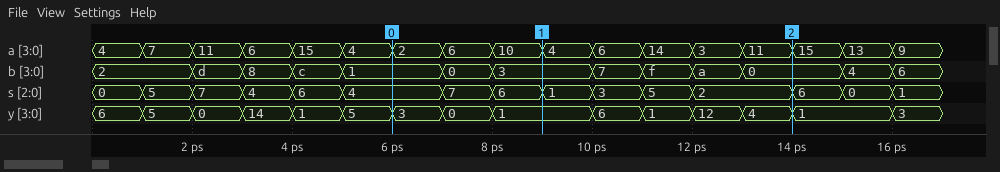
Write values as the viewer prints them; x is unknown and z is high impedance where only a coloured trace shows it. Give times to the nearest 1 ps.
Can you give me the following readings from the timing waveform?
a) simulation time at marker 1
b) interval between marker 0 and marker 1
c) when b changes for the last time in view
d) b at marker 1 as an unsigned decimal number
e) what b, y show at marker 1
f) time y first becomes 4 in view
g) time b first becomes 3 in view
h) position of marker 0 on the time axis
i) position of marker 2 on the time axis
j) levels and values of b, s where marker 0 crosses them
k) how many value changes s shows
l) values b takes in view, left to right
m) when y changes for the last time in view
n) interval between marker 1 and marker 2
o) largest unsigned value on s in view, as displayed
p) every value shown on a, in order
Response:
9 ps
3 ps
16 ps
3
b=3, y=1
13 ps
8 ps
6 ps
14 ps
b=1, s=4
14
2, d, 8, c, 1, 0, 3, 7, f, a, 0, 4, 6
16 ps
5 ps
7
4, 7, 11, 6, 15, 4, 2, 6, 10, 4, 6, 14, 3, 11, 15, 13, 9
